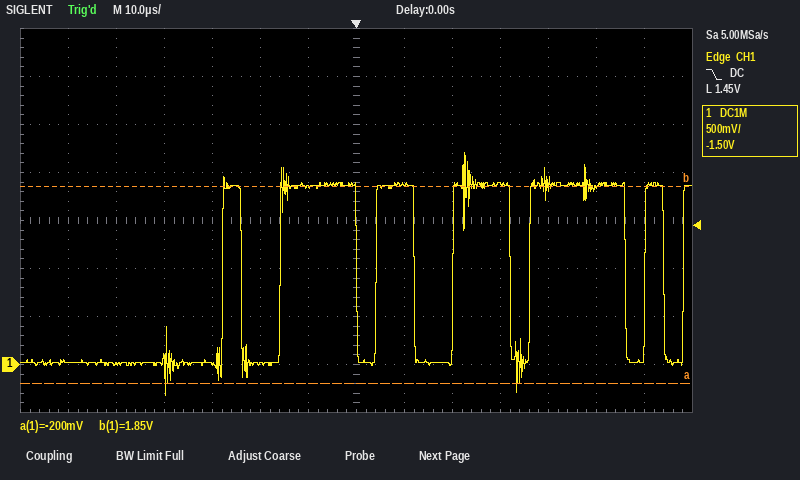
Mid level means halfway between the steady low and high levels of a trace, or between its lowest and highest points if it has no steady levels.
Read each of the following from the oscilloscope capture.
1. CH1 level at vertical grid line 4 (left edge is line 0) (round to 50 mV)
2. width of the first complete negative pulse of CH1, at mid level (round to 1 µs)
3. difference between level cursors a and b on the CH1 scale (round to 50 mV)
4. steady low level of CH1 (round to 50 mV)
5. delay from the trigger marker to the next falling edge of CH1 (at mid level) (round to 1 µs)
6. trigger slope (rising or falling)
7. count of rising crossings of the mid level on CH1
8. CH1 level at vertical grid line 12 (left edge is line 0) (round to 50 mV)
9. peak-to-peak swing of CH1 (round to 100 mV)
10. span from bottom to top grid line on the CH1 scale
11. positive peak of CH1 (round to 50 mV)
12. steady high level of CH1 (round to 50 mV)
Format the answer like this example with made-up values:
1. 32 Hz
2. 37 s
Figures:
1. 0 mV
2. 8 µs
3. 2.05 V
4. 0 mV
5. 12 µs
6. falling
7. 7
8. 1.85 V
9. 2.50 V
10. 4 V
11. 2.20 V
12. 1.85 V
